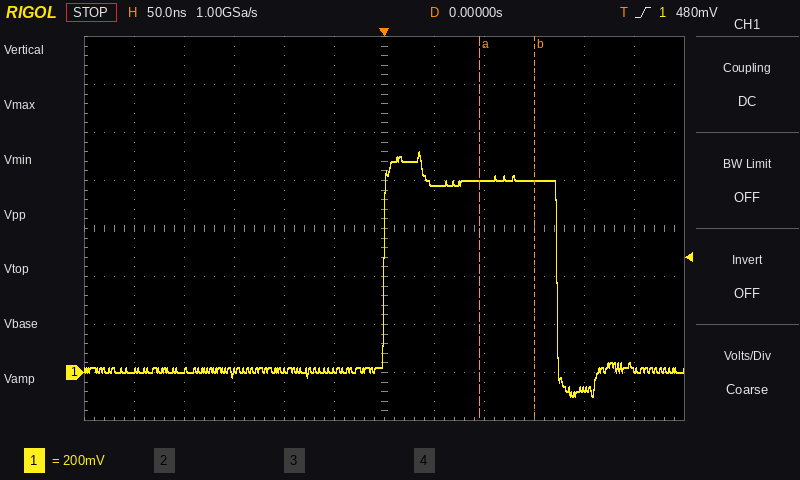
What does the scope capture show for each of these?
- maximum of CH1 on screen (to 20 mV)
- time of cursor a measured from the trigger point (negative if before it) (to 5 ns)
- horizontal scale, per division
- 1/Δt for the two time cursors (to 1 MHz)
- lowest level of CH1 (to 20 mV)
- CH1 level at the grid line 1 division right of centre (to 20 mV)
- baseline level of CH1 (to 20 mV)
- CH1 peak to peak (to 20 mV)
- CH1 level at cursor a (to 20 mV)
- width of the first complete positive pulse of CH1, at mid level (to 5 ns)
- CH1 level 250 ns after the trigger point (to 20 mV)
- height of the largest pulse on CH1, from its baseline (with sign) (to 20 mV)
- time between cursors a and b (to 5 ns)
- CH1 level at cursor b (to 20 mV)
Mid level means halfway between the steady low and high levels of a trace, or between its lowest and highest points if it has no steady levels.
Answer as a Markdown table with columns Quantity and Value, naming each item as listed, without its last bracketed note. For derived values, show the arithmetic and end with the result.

| Quantity | Value |
|---|---|
| maximum of CH1 on screen | 920 mV |
| time of cursor a measured from the trigger point (negative if before it) | +95 ns |
| horizontal scale, per division | 50 ns |
| 1/Δt for the two time cursors | 1 / 55 ns ≈ 18 MHz |
| lowest level of CH1 | -100 mV |
| CH1 level at the grid line 1 division right of centre | 780 mV |
| baseline level of CH1 | 0 mV |
| CH1 peak to peak | 920 mV − (-100 mV) = 1.02 V |
| CH1 level at cursor a | 800 mV |
| width of the first complete positive pulse of CH1, at mid level | 175 ns |
| CH1 level 250 ns after the trigger point | 20 mV |
| height of the largest pulse on CH1, from its baseline (with sign) | 920 mV − (0 mV) = +920 mV |
| time between cursors a and b | 55 ns |
| CH1 level at cursor b | 800 mV |
